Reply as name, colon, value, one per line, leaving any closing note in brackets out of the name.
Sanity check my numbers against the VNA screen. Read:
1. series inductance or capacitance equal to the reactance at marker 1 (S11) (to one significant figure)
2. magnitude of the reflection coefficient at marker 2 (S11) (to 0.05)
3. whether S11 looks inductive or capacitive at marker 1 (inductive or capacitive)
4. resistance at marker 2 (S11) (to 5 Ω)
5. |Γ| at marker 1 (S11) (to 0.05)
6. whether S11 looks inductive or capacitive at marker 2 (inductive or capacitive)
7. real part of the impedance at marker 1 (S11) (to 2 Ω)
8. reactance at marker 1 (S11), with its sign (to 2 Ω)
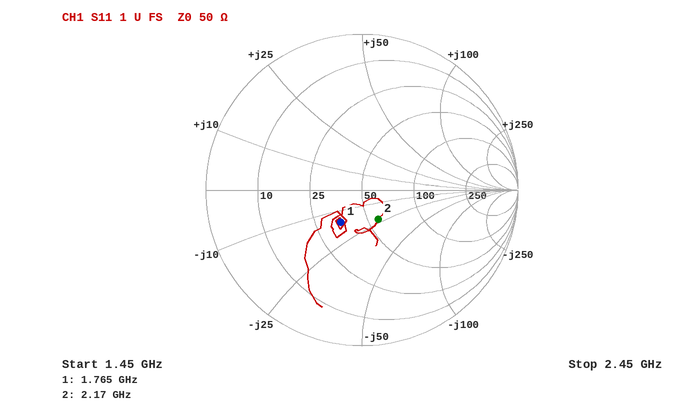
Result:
series inductance or capacitance equal to the reactance at marker 1 (S11): 6 pF
magnitude of the reflection coefficient at marker 2 (S11): 0.20
whether S11 looks inductive or capacitive at marker 1: capacitive
resistance at marker 2 (S11): 55 Ω
|Γ| at marker 1 (S11): 0.25
whether S11 looks inductive or capacitive at marker 2: capacitive
real part of the impedance at marker 1 (S11): 36 Ω
reactance at marker 1 (S11), with its sign: -16 Ω
